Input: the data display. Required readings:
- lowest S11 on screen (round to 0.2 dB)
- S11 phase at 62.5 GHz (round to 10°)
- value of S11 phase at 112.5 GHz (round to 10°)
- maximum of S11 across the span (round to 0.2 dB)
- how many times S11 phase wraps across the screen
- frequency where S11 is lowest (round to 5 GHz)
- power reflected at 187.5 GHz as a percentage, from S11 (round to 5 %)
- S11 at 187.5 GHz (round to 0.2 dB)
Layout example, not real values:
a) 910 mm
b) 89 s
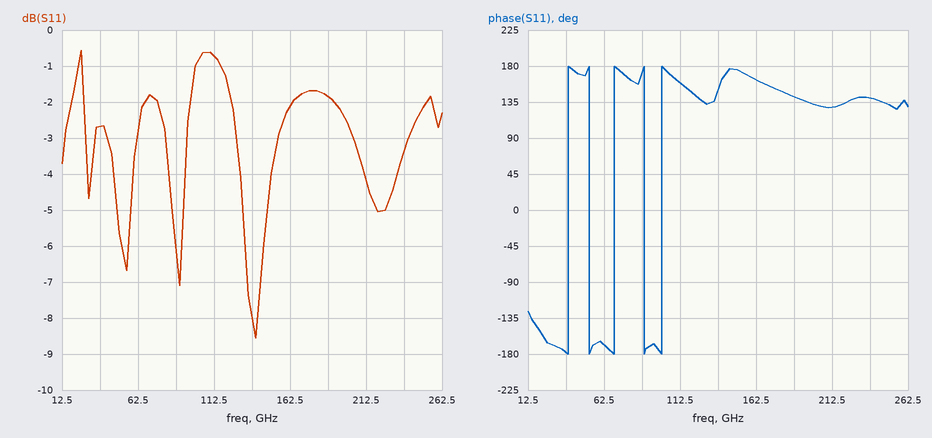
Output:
a) -8.6 dB
b) -170°
c) 160°
d) -0.6 dB
e) 5
f) 140 GHz
g) 65 %
h) -1.8 dB
